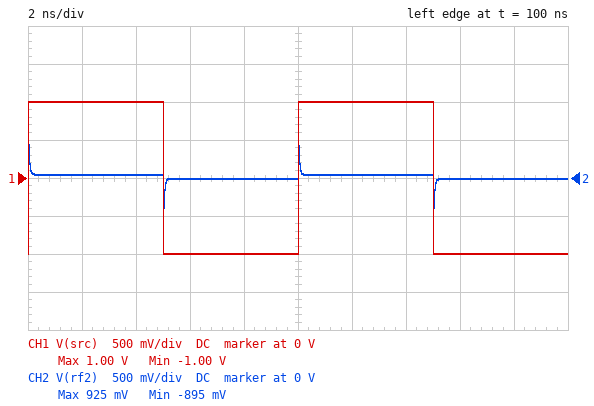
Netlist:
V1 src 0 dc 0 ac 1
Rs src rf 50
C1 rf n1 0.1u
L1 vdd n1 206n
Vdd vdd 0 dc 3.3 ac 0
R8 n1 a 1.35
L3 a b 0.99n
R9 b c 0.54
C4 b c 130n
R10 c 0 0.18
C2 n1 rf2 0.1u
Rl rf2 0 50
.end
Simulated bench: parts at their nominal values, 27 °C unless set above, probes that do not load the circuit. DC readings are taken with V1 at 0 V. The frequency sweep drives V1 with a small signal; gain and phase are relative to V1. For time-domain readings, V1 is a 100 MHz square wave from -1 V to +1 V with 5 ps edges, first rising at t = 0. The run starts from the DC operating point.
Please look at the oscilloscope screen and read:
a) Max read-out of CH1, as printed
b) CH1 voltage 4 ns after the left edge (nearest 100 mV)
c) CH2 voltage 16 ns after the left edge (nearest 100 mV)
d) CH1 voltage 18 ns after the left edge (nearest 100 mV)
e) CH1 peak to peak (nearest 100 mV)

1.00 V
1.0 V
0 V
-1.0 V
2.0 V
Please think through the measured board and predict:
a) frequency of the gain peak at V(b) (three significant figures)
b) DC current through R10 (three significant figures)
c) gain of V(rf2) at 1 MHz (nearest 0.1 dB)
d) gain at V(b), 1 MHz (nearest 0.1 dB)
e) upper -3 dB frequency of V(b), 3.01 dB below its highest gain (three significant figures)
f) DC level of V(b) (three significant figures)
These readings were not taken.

1.91 MHz
1.59 A
-33.1 dB
-42.6 dB
4.84 MHz
1.15 V
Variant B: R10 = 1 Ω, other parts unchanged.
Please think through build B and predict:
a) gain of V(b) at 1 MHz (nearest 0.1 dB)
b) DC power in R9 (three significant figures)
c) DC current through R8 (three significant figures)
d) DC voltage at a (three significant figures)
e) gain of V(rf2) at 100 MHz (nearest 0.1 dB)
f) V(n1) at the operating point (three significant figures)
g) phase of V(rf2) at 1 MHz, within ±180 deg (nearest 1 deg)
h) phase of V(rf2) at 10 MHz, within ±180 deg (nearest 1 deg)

-38.2 dB
704 mW
1.14 A
1.76 V
-27.1 dB
3.30 V
66 deg
9 deg
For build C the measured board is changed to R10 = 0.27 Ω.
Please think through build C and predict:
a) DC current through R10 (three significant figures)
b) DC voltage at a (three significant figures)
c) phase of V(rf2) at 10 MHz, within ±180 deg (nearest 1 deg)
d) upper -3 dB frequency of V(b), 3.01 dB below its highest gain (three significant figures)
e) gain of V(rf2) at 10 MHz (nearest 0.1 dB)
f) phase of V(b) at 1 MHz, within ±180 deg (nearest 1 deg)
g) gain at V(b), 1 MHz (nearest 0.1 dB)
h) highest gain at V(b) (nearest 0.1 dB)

1.53 A
1.24 V
5 deg
5.74 MHz
-30.2 dB
46 deg
-41.9 dB
-39.8 dB
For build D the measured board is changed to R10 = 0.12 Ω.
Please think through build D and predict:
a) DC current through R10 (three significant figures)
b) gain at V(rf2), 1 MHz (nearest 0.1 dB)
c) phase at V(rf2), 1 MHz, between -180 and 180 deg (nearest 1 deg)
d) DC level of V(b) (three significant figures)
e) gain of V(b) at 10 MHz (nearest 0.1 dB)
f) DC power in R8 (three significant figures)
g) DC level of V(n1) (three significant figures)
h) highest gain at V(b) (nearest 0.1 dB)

1.64 A
-33.2 dB
56 deg
1.08 V
-49.1 dB
3.64 W
3.30 V
-41.5 dB
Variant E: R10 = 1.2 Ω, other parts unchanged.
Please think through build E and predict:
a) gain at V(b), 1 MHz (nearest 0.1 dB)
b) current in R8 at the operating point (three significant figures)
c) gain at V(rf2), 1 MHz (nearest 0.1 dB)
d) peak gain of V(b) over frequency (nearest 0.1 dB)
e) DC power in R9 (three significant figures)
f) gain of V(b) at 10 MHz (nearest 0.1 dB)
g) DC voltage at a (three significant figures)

-37.6 dB
1.07 A
-32.4 dB
-32.9 dB
616 mW
-33.1 dB
1.86 V
